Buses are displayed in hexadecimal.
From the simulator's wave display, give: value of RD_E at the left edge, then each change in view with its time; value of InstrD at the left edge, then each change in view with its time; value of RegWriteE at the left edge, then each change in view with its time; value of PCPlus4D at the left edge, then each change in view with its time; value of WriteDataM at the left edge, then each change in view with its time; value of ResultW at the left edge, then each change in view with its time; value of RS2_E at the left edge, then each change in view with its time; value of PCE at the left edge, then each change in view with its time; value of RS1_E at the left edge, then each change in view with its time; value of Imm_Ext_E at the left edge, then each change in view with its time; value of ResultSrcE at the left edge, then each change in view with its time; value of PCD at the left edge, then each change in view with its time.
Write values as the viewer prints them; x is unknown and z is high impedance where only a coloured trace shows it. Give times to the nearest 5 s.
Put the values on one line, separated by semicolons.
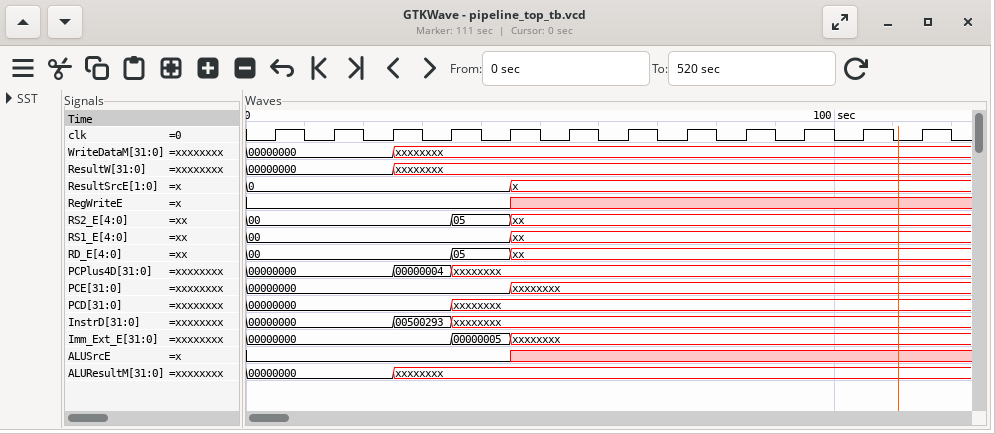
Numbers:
00, 05 at 35 s, xx at 45 s; 00000000, 00500293 at 25 s, xxxxxxxx at 35 s; 0, x at 45 s; 00000000, 00000004 at 25 s, xxxxxxxx at 35 s; 00000000, xxxxxxxx at 25 s; 00000000, xxxxxxxx at 25 s; 00, 05 at 35 s, xx at 45 s; 00000000, xxxxxxxx at 45 s; 00, xx at 45 s; 00000000, 00000005 at 35 s, xxxxxxxx at 45 s; 0, x at 45 s; 00000000, xxxxxxxx at 35 s
